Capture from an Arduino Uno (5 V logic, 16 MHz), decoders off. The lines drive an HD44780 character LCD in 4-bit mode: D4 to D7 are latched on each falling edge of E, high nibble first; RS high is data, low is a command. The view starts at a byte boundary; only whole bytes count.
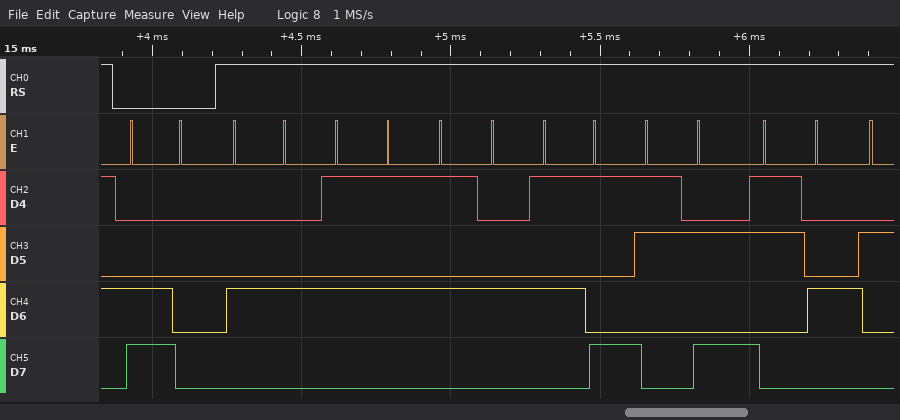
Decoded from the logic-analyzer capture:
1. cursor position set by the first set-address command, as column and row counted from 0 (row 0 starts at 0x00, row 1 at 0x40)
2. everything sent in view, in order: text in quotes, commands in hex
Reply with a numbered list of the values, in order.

1. column 0, row 1
2. 0xC0 "DUTY:4"
